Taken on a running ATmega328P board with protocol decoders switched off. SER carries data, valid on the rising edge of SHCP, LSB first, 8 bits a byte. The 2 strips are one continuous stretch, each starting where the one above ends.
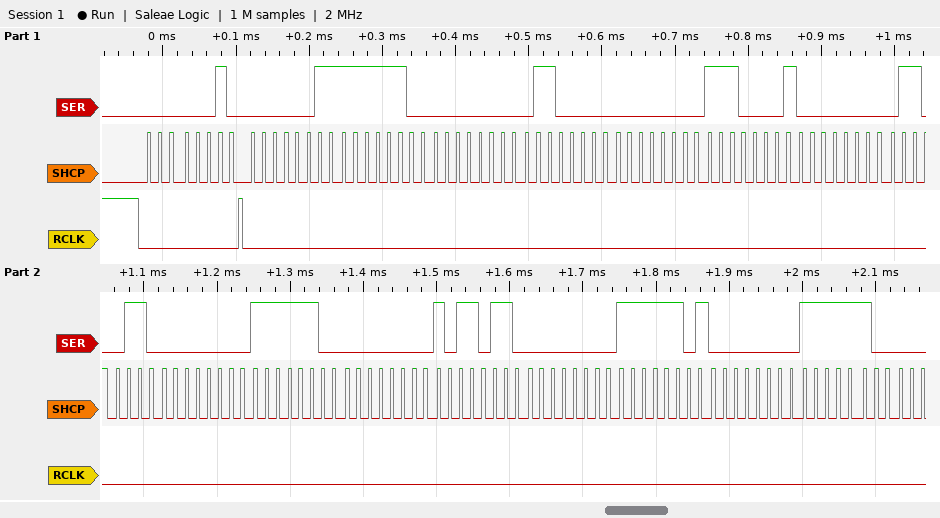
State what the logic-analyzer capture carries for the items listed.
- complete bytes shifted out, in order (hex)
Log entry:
40 C0 3F 00 06 00 87 00 66 00 3F 00 6D 00 BF 00 3F
